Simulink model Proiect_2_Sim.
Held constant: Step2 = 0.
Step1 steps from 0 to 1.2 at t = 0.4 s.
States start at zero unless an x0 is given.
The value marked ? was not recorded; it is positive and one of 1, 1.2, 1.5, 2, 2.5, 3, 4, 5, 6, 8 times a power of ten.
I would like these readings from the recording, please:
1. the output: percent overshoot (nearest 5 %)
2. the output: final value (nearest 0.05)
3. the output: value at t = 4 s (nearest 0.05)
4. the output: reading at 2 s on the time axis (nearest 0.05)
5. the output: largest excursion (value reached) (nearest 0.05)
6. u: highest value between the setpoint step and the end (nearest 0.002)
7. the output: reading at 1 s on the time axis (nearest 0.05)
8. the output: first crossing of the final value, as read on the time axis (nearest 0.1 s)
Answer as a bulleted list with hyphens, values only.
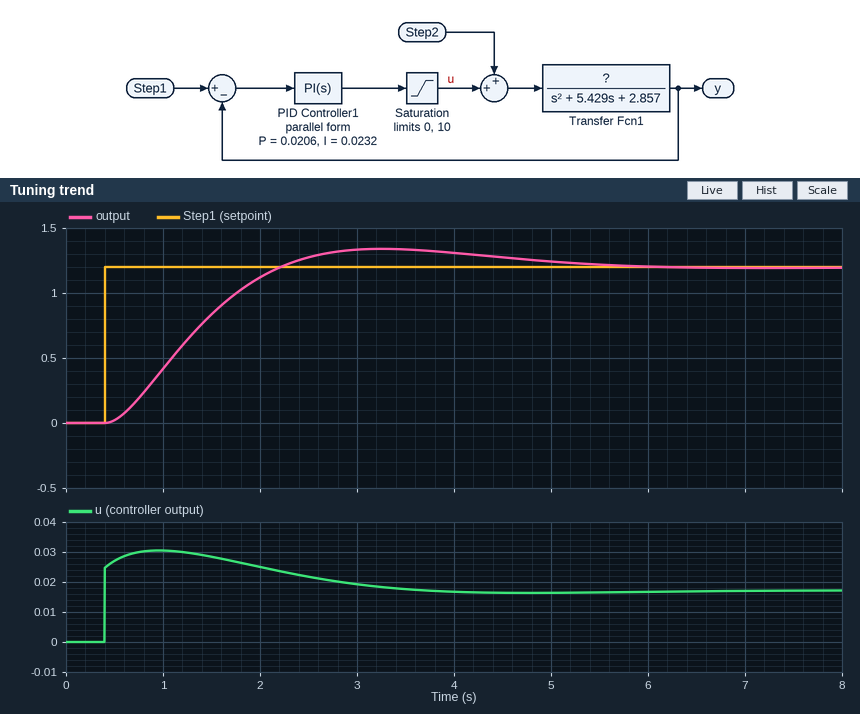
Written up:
- 10 %
- 1.20
- 1.30
- 1.10
- 1.35
- 0.030
- 0.40
- 2.2 s
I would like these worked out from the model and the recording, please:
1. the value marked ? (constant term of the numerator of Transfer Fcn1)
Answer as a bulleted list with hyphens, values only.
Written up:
- 200
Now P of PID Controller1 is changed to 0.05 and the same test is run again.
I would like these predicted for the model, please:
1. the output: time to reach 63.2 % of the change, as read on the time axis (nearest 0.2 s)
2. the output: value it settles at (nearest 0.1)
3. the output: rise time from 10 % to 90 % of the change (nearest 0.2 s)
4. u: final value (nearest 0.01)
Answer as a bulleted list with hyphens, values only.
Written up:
- 1.0 s
- 1.2
- 0.8 s
- 0.02
